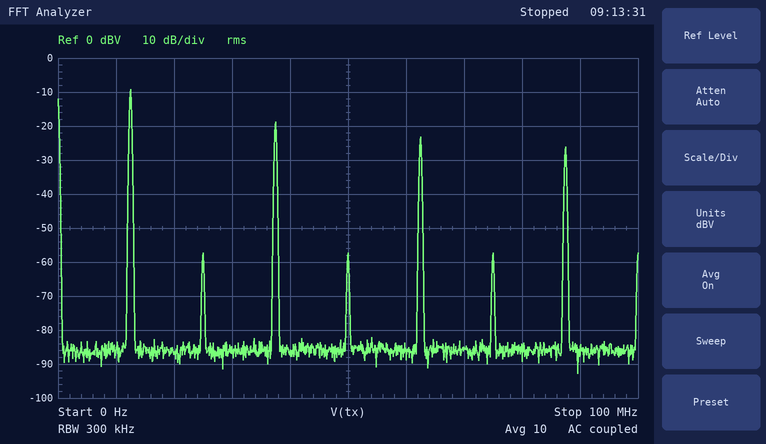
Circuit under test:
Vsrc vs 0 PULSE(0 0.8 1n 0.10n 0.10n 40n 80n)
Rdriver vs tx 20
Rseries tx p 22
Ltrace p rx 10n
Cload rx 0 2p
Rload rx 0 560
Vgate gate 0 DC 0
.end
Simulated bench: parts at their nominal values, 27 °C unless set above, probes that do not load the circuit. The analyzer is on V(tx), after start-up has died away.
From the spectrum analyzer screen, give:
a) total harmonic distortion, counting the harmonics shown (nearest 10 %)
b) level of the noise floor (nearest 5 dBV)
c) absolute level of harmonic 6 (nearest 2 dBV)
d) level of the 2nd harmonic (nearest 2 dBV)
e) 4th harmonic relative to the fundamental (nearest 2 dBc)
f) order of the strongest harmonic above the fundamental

40 %
-85 dBV
-58 dBV
-58 dBV
-48 dBc
3
